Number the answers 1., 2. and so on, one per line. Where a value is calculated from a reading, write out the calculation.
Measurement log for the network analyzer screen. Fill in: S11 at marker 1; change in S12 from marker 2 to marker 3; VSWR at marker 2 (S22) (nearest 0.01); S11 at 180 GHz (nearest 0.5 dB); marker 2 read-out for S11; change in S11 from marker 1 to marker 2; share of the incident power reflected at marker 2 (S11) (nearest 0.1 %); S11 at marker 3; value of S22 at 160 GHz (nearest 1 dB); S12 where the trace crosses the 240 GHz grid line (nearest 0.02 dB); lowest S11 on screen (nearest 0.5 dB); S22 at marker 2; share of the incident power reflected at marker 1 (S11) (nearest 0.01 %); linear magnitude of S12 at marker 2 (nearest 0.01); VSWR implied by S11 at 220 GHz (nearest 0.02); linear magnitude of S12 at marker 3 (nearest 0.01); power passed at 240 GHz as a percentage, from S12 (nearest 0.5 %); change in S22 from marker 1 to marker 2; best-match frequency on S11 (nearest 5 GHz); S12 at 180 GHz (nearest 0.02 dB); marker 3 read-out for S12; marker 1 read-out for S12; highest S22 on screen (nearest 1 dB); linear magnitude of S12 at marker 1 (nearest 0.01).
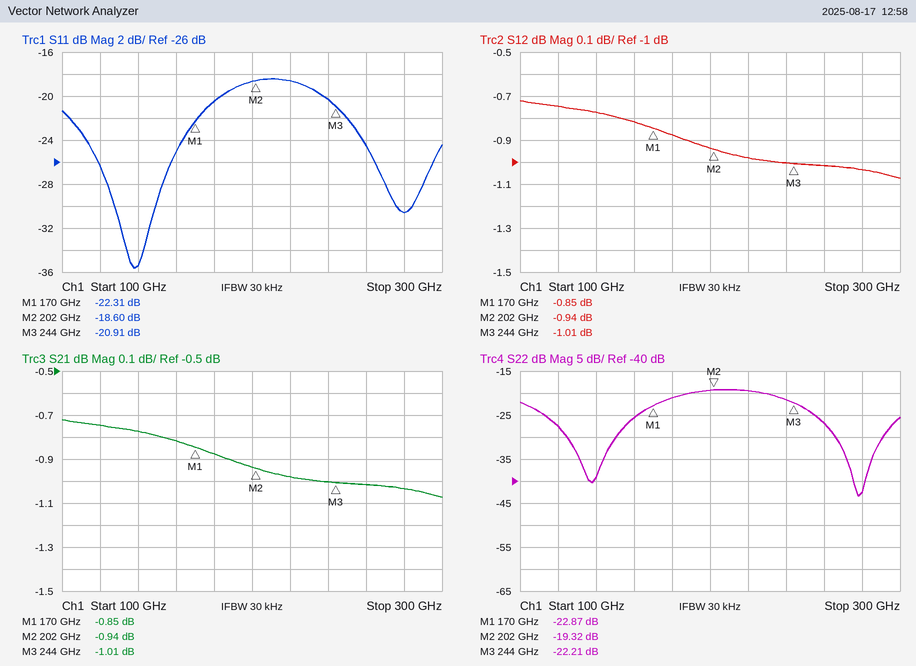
1. -22.31 dB
2. -1.01 − (-0.94) = -0.07 dB
3. (1 + 0.1081)/(1 − 0.1081) ≈ 1.24
4. -20.5 dB
5. -18.60 dB
6. -18.6 − (-22.31) = 3.71 dB
7. 10^(-18.6/10) ≈ 1.4 %
8. -20.91 dB
9. -26 dB
10. -1.00 dB
11. -35.5 dB
12. -19.32 dB
13. 10^(-22.31/10) ≈ 0.59 %
14. 10^(-0.94/20) ≈ 0.90
15. |Γ| = 10^(-18.5/20) = 0.1189; VSWR = (1 + 0.1189)/(1 − 0.1189) ≈ 1.27, so 1.26 to the nearest 0.02
16. 10^(-1.01/20) ≈ 0.89
17. 10^(-1/10) ≈ 79.4 %, so 79.5 % to the nearest 0.5 %
18. -19.32 − (-22.87) = 3.55 dB
19. 140 GHz
20. -0.88 dB
21. -1.01 dB
22. -0.85 dB
23. -19 dB
24. 10^(-0.85/20) ≈ 0.91
